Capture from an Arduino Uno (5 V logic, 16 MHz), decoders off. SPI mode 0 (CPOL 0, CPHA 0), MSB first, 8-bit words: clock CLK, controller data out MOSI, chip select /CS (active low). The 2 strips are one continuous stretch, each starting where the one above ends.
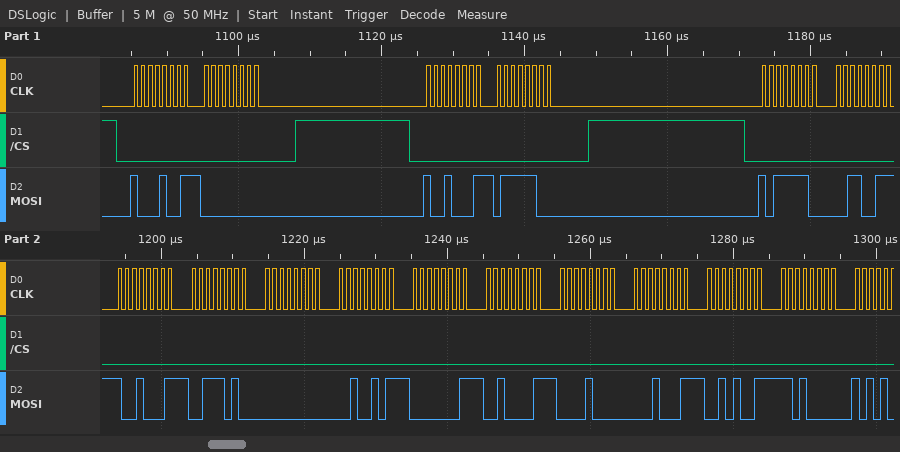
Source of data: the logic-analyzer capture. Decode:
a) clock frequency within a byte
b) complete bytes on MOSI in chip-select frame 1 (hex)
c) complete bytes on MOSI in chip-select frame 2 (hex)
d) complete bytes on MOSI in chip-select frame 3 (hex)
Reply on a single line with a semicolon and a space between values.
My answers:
1 MHz; 89 00; 91 7C; BE 33 91 3A 00 25 01 21 08 11 29 D0
